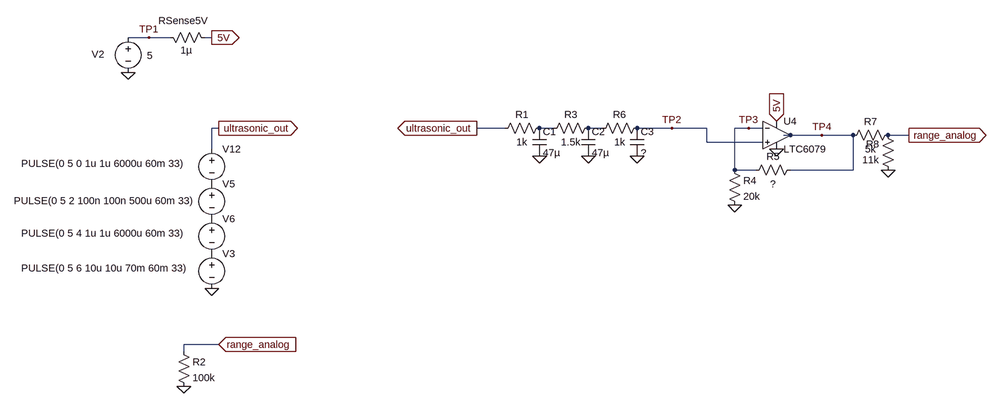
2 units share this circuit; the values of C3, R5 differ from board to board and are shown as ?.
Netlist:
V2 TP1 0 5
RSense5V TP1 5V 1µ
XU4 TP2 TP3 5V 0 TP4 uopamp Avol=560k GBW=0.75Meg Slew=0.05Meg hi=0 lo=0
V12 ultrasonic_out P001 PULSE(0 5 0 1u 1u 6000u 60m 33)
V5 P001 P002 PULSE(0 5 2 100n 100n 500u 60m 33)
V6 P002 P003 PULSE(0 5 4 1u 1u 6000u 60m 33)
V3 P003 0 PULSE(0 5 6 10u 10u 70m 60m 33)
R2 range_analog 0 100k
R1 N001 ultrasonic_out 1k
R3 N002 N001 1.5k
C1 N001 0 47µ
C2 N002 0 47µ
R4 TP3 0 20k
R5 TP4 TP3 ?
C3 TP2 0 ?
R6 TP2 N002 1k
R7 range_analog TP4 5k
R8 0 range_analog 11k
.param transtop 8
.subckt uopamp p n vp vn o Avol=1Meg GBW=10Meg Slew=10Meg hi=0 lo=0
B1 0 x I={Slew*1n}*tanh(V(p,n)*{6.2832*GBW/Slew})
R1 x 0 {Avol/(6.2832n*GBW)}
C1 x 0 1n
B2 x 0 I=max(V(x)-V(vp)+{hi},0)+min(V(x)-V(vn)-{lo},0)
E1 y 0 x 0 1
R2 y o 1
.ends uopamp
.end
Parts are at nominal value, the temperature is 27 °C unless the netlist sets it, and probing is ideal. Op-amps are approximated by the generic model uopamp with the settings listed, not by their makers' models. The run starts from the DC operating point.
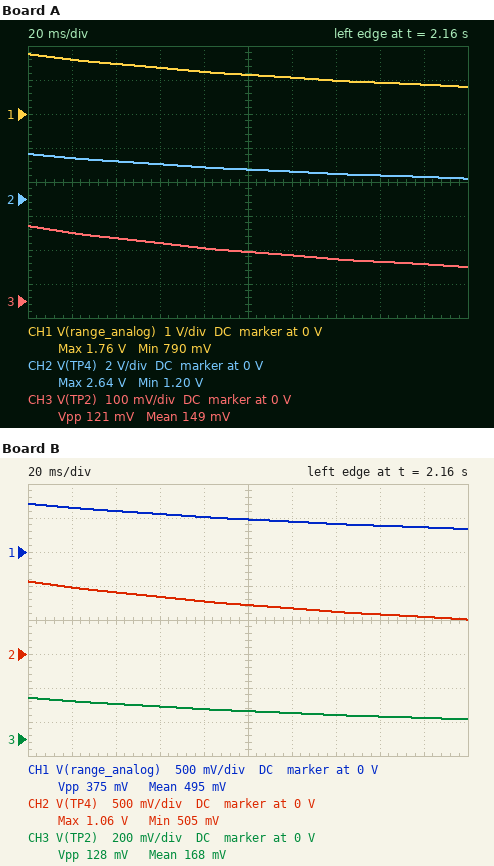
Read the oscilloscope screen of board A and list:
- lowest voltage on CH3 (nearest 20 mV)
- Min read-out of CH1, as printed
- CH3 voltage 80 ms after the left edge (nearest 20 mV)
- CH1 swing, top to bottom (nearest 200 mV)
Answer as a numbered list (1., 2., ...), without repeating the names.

1. 100 mV
2. 790 mV
3. 160 mV
4. 1.0 V
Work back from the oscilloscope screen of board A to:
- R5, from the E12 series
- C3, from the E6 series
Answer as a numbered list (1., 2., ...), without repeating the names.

1. 220 kΩ
2. 15 µF
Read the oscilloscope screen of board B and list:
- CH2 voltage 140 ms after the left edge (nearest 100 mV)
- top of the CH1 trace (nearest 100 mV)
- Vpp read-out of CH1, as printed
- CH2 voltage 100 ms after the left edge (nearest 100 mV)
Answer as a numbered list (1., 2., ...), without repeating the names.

1. 600 mV
2. 700 mV
3. 375 mV
4. 700 mV
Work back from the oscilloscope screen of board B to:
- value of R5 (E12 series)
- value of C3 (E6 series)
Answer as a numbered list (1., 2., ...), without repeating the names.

1. 68 kΩ
2. 22 µF
